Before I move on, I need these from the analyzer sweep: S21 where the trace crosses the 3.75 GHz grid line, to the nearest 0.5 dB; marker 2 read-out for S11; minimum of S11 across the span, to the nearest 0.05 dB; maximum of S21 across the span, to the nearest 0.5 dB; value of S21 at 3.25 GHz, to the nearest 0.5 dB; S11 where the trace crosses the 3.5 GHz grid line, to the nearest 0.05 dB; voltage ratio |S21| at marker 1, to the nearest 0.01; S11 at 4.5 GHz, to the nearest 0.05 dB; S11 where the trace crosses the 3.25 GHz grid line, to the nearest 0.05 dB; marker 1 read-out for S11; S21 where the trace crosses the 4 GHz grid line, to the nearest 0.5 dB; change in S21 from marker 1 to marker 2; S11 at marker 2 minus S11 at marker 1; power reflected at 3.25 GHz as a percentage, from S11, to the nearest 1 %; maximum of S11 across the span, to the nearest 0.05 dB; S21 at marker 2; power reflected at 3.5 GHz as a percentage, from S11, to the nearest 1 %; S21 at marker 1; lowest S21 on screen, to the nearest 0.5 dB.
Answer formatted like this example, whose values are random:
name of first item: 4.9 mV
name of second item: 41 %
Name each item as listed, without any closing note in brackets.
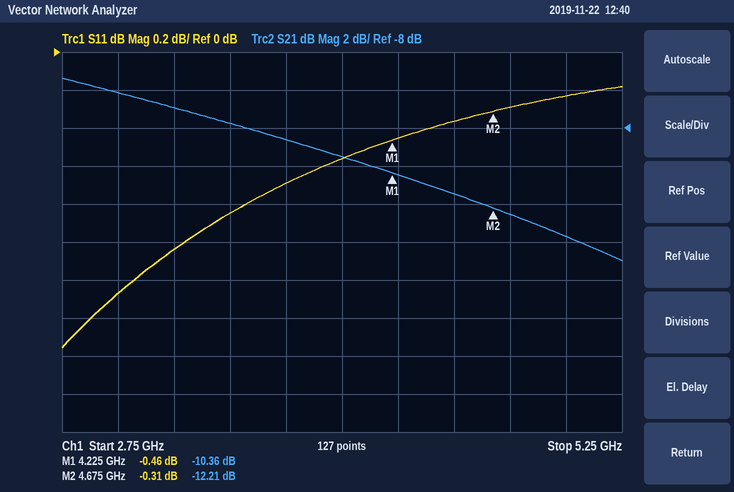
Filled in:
S21 where the trace crosses the 3.75 GHz grid line, to the nearest 0.5 dB: -8.5 dB
marker 2 read-out for S11: -0.31 dB
minimum of S11 across the span, to the nearest 0.05 dB: -1.55 dB
maximum of S21 across the span, to the nearest 0.5 dB: -5.5 dB
value of S21 at 3.25 GHz, to the nearest 0.5 dB: -7.0 dB
S11 where the trace crosses the 3.5 GHz grid line, to the nearest 0.05 dB: -0.85 dB
voltage ratio |S21| at marker 1, to the nearest 0.01: 0.30
S11 at 4.5 GHz, to the nearest 0.05 dB: -0.35 dB
S11 where the trace crosses the 3.25 GHz grid line, to the nearest 0.05 dB: -1.05 dB
marker 1 read-out for S11: -0.46 dB
S21 where the trace crosses the 4 GHz grid line, to the nearest 0.5 dB: -9.5 dB
change in S21 from marker 1 to marker 2: -1.85 dB
S11 at marker 2 minus S11 at marker 1: 0.15 dB
power reflected at 3.25 GHz as a percentage, from S11, to the nearest 1 %: 79 %
maximum of S11 across the span, to the nearest 0.05 dB: -0.20 dB
S21 at marker 2: -12.21 dB
power reflected at 3.5 GHz as a percentage, from S11, to the nearest 1 %: 82 %
S21 at marker 1: -10.36 dB
lowest S21 on screen, to the nearest 0.5 dB: -15.0 dB
